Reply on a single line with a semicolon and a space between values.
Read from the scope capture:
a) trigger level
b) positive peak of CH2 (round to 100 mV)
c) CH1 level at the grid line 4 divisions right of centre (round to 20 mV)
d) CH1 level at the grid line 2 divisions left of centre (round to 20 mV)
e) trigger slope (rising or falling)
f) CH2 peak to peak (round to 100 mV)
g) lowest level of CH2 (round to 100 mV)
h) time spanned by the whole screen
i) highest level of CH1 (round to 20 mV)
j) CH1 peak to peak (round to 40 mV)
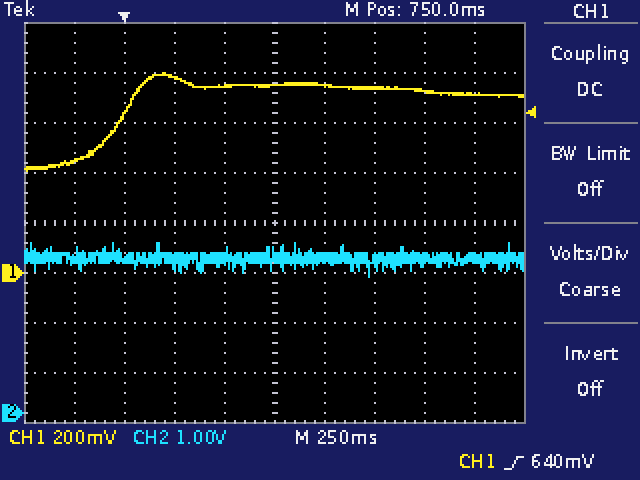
640 mV; 3.4 V; 720 mV; 780 mV; rising; 700 mV; 2.7 V; 2.5 s; 800 mV; 400 mV
